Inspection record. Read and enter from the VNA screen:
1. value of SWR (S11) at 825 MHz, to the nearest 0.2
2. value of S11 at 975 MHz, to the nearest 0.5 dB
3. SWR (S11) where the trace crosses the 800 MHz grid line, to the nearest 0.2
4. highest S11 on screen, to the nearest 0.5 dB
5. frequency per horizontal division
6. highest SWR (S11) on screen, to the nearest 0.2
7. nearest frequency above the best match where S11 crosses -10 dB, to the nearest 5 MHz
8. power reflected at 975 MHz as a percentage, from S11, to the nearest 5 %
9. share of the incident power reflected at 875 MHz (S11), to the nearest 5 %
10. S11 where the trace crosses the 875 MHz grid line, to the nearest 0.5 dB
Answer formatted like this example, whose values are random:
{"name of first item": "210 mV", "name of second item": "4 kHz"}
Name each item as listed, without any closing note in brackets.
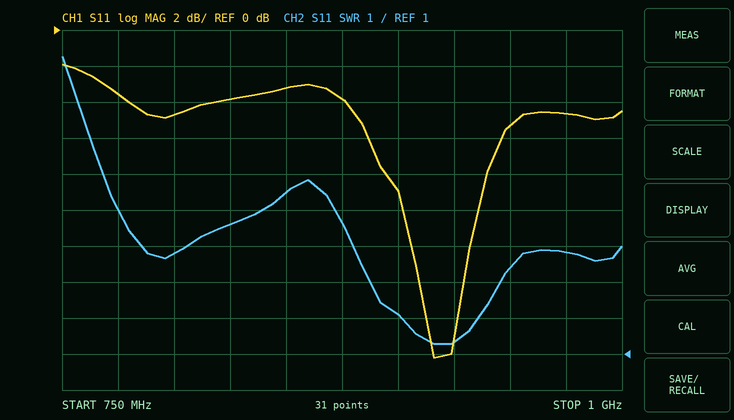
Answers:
{"value of SWR (S11) at 825 MHz, to the nearest 0.2": "4.6", "value of S11 at 975 MHz, to the nearest 0.5 dB": "-4.5 dB", "SWR (S11) where the trace crosses the 800 MHz grid line, to the nearest 0.2": "3.8", "highest S11 on screen, to the nearest 0.5 dB": "-2.0 dB", "frequency per horizontal division": "25 MHz", "highest SWR (S11) on screen, to the nearest 0.2": "9.2", "nearest frequency above the best match where S11 crosses -10 dB, to the nearest 5 MHz": "935 MHz", "power reflected at 975 MHz as a percentage, from S11, to the nearest 5 %": "35 %", "share of the incident power reflected at 875 MHz (S11), to the nearest 5 %": "40 %", "S11 where the trace crosses the 875 MHz grid line, to the nearest 0.5 dB": "-4.0 dB"}
